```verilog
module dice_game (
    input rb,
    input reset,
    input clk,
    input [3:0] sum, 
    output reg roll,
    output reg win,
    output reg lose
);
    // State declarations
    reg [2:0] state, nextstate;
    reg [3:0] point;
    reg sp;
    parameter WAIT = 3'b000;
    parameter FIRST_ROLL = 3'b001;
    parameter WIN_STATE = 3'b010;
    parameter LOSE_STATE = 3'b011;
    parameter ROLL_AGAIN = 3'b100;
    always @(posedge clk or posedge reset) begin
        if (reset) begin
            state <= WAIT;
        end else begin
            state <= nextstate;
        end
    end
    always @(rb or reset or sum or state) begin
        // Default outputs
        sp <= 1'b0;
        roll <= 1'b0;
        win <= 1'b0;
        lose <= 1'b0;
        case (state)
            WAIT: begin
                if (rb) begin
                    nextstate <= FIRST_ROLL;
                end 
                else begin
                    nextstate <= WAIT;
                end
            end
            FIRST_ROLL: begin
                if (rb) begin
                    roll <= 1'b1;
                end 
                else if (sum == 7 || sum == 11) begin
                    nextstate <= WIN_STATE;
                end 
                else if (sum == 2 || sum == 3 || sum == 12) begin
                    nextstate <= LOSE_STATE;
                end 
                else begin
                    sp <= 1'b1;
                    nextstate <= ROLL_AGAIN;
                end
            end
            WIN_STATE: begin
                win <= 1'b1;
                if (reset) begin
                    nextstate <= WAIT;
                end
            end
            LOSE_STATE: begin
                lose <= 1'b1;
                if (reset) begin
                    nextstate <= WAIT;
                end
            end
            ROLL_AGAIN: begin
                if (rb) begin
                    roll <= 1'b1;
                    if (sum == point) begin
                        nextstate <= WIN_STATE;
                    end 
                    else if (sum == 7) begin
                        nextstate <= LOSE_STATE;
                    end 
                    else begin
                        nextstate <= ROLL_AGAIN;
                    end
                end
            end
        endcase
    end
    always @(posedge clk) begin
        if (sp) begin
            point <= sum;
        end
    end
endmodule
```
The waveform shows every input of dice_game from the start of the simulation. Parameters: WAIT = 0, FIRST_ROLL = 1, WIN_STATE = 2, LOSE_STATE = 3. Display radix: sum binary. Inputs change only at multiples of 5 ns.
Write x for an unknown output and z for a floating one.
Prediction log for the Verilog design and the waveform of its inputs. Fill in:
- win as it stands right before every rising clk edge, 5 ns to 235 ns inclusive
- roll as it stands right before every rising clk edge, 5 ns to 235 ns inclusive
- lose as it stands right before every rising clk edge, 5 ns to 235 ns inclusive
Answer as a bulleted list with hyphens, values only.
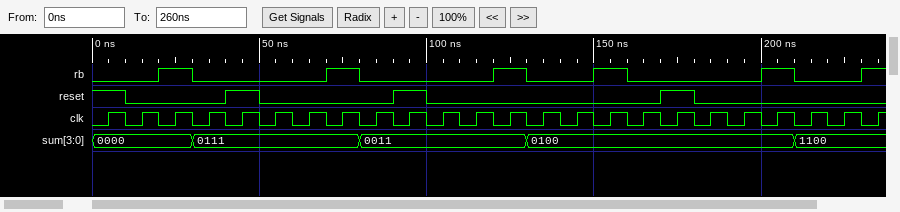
- 0 0 0 0 0 0 0 0 0 0 0 0 0 0 0 0 1 0 0 0 0 0 0 0
- 0 0 0 0 0 0 0 0 0 0 0 0 0 0 0 1 0 0 0 0 0 0 0 0
- 0 0 0 0 0 0 0 0 0 0 0 0 0 0 0 0 0 0 0 0 0 0 1 1
